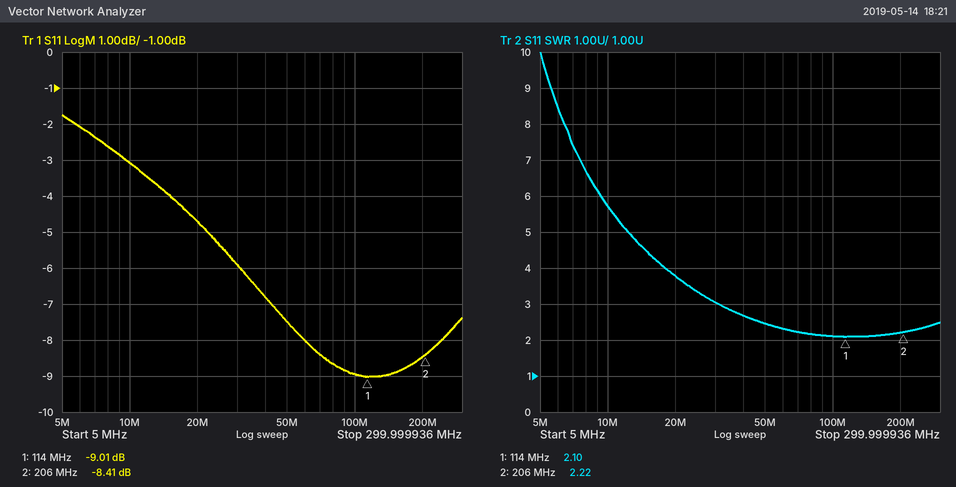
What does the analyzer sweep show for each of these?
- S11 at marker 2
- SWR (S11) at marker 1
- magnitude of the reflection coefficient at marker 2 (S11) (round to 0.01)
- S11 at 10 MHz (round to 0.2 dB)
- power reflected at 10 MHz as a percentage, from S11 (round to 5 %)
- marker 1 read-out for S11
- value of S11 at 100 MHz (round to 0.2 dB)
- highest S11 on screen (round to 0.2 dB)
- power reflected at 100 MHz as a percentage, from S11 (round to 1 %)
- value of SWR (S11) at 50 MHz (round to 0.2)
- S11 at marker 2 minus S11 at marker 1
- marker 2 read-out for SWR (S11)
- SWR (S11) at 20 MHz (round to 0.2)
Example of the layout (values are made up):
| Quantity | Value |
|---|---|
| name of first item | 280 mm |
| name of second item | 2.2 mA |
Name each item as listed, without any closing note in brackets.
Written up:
| Quantity | Value |
|---|---|
| S11 at marker 2 | -8.41 dB |
| SWR (S11) at marker 1 | 2.10 |
| magnitude of the reflection coefficient at marker 2 (S11) | 0.38 |
| S11 at 10 MHz | -3.0 dB |
| power reflected at 10 MHz as a percentage, from S11 | 50 % |
| marker 1 read-out for S11 | -9.01 dB |
| value of S11 at 100 MHz | -9.0 dB |
| highest S11 on screen | -1.8 dB |
| power reflected at 100 MHz as a percentage, from S11 | 13 % |
| value of SWR (S11) at 50 MHz | 2.4 |
| S11 at marker 2 minus S11 at marker 1 | 0.60 dB |
| marker 2 read-out for SWR | 2.22 |
| SWR (S11) at 20 MHz | 3.8 |
